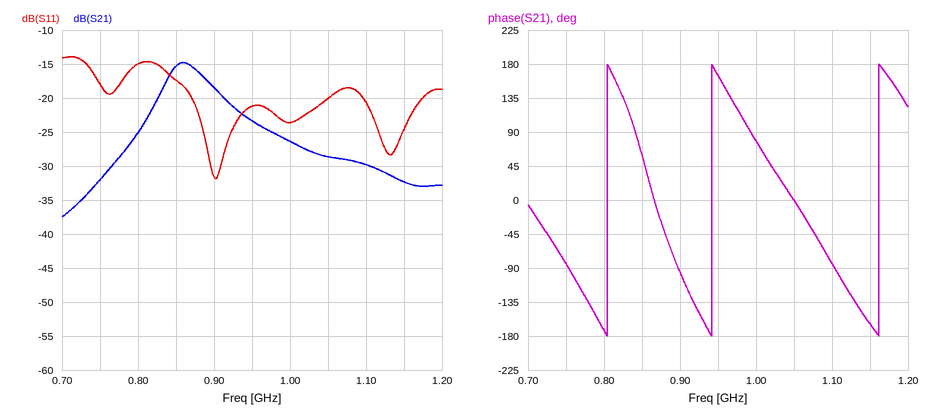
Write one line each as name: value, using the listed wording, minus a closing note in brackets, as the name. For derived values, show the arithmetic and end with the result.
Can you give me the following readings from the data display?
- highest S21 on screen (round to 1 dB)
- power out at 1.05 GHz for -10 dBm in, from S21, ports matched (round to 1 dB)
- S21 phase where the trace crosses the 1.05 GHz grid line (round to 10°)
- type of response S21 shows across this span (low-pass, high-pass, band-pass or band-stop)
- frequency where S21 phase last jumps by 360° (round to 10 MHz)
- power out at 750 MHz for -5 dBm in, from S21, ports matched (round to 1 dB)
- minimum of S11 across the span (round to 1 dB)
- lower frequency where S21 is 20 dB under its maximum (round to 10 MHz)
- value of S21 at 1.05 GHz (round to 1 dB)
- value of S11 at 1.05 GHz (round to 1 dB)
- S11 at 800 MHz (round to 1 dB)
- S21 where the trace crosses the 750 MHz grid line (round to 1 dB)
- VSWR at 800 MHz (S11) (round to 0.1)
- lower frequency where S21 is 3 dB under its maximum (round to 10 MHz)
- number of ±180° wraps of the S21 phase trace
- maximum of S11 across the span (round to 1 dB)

highest S21 on screen: -15 dB
power out at 1.05 GHz for -10 dBm in, from S21, ports matched: -10 dBm + (-29 dB) = -39 dBm
S21 phase where the trace crosses the 1.05 GHz grid line: 0°
type of response S21 shows across this span: band-pass
frequency where S21 phase last jumps by 360°: 1.16 GHz
power out at 750 MHz for -5 dBm in, from S21, ports matched: -5 dBm + (-32 dB) = -37 dBm
minimum of S11 across the span: -32 dB
lower frequency where S21 is 20 dB under its maximum: 730 MHz
value of S21 at 1.05 GHz: -29 dB
value of S11 at 1.05 GHz: -20 dB
S11 at 800 MHz: -15 dB
S21 where the trace crosses the 750 MHz grid line: -32 dB
VSWR at 800 MHz (S11): |Γ| = 10^(-15/20) = 0.1778; VSWR = (1 + 0.1778)/(1 − 0.1778) ≈ 1.4
lower frequency where S21 is 3 dB under its maximum: 840 MHz
number of ±180° wraps of the S21 phase trace: 3
maximum of S11 across the span: -14 dB
